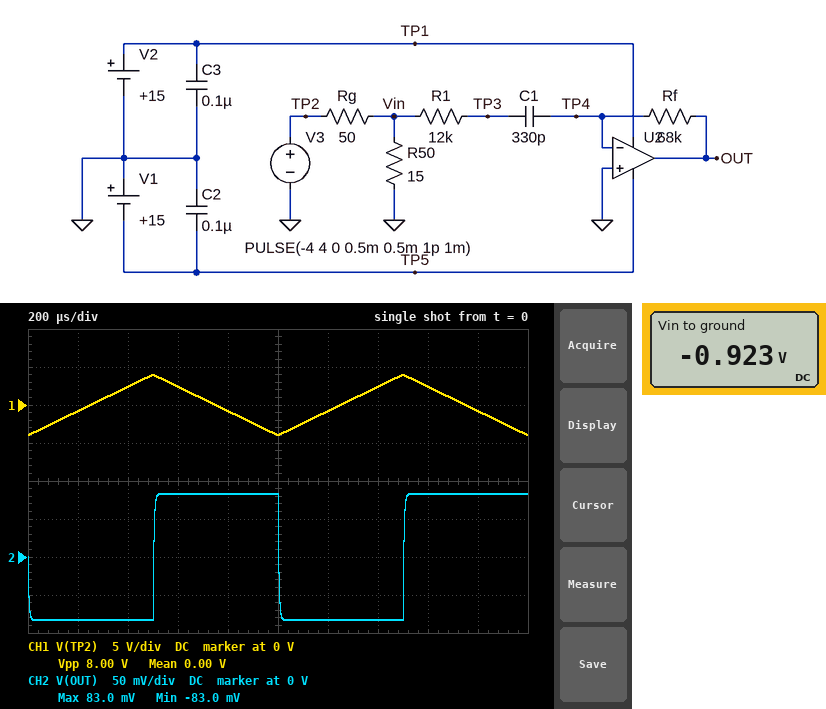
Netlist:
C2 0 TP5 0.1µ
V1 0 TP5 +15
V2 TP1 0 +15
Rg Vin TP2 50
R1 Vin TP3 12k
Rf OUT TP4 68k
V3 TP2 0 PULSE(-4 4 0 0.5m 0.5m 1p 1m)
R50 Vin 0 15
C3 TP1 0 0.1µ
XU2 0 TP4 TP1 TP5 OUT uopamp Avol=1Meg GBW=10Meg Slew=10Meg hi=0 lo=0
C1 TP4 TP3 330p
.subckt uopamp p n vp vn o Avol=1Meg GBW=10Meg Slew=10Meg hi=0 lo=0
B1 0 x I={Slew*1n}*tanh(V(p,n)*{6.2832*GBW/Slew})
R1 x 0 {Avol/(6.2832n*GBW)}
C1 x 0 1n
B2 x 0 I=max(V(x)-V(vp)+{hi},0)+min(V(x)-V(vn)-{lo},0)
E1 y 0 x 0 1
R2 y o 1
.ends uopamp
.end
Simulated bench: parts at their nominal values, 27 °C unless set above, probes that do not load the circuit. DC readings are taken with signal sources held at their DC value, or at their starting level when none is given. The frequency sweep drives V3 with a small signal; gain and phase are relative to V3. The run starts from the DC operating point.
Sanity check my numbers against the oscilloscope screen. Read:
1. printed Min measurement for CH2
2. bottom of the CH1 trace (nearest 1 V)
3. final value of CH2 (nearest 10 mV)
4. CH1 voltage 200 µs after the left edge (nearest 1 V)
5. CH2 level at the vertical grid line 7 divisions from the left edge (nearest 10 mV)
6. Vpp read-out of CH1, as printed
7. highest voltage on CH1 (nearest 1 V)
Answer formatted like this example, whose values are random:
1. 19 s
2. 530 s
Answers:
1. -83.0 mV
2. -4 V
3. 80 mV
4. -1 V
5. -80 mV
6. 8.00 V
7. 4 V
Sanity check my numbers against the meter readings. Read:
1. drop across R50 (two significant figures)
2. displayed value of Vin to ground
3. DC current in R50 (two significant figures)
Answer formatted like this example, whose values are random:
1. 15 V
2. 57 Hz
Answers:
1. 920 mV
2. -0.923 V
3. 62 mA
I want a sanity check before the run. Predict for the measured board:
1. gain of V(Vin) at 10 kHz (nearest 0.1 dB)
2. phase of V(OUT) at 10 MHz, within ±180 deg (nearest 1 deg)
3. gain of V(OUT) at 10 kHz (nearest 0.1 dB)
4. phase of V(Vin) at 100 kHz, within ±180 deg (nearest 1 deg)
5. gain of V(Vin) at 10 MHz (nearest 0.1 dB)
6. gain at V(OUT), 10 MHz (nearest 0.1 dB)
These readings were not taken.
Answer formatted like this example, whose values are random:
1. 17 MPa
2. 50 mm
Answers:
1. -12.7 dB
2. 99 deg
3. -10.0 dB
4. 0 deg
5. -12.7 dB
6. -14.2 dB
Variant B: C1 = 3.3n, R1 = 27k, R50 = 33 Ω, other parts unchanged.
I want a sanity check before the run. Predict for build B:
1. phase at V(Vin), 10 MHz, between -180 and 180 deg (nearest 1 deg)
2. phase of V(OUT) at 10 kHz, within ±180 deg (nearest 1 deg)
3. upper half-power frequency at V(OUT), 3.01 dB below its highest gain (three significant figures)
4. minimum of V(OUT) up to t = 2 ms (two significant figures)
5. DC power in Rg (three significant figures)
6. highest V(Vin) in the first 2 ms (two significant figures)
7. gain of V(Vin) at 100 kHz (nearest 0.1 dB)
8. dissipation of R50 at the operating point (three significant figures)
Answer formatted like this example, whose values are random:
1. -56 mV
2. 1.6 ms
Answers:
1. 0 deg
2. -170 deg
3. 2.85 MHz
4. -1.4 V
5. 116 mW
6. 1.6 V
7. -8.0 dB
8. 76.6 mW
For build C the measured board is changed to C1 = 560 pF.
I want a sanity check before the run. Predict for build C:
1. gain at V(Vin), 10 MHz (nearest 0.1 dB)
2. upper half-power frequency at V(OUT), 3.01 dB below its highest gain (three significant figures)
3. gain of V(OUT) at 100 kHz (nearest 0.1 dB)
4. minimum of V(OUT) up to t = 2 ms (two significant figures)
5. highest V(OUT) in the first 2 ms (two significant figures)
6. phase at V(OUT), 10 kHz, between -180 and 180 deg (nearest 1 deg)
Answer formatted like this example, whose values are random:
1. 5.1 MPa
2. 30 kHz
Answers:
1. -12.7 dB
2. 1.53 MHz
3. 2.2 dB
4. -140 mV
5. 140 mV
6. -113 deg
